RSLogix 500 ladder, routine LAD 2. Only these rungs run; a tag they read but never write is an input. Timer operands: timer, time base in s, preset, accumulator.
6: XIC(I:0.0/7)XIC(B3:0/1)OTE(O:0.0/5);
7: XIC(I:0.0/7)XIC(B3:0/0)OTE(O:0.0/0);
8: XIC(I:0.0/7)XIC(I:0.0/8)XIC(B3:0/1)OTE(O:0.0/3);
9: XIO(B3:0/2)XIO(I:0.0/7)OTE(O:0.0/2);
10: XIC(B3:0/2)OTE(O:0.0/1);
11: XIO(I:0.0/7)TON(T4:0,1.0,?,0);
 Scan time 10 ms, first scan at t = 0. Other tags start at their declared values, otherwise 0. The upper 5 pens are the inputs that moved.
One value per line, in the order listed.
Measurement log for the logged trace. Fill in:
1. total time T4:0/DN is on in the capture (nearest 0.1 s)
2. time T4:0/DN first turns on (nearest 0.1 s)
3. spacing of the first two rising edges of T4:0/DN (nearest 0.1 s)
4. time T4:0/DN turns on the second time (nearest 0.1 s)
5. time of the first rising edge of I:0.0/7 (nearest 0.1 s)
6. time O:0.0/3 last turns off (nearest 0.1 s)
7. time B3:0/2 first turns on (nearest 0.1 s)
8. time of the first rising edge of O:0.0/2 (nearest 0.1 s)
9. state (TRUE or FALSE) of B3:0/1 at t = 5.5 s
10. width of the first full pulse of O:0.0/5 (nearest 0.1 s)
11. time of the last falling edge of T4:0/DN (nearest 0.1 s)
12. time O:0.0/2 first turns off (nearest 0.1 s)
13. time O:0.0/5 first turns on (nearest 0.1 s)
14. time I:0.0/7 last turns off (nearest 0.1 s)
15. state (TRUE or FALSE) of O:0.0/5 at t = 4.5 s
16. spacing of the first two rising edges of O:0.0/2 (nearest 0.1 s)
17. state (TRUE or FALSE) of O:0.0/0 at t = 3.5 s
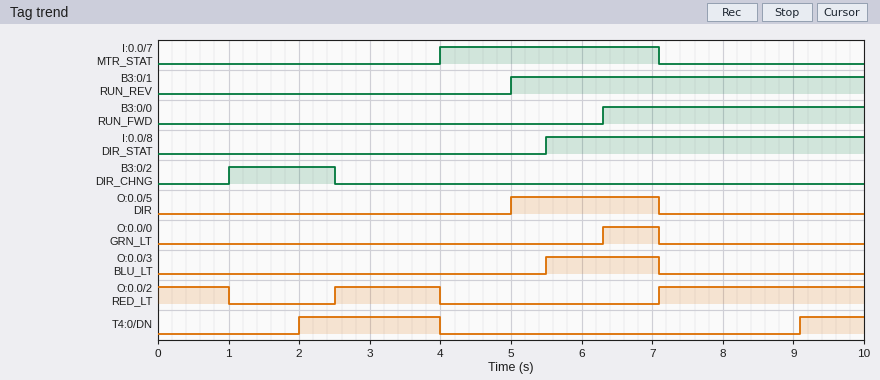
2.9 s
2.0 s
7.1 s
9.1 s
4.0 s
7.1 s
1.0 s
2.5 s
TRUE
2.1 s
4.0 s
1.0 s
5.0 s
7.1 s
FALSE
4.6 s
FALSE
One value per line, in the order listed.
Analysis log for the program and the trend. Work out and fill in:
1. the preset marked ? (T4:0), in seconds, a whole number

2 s
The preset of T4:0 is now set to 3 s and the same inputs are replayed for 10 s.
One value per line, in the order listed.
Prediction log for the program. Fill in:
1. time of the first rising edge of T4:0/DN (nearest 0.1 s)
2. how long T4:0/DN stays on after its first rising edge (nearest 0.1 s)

3.0 s
1.0 s
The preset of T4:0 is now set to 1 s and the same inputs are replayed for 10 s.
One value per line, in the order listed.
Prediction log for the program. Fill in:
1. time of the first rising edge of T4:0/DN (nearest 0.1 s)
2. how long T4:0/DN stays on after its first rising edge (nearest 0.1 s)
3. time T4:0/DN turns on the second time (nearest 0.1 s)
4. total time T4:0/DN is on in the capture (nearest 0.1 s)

1.0 s
3.0 s
8.1 s
4.9 s
